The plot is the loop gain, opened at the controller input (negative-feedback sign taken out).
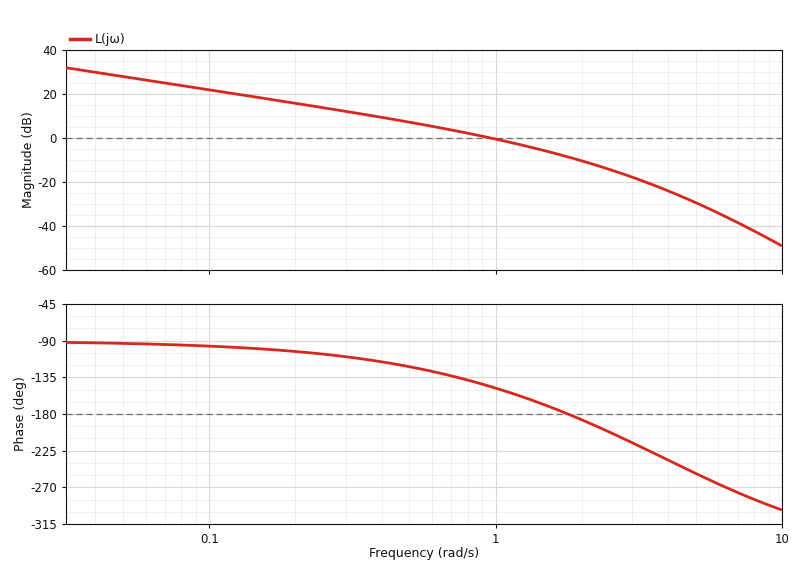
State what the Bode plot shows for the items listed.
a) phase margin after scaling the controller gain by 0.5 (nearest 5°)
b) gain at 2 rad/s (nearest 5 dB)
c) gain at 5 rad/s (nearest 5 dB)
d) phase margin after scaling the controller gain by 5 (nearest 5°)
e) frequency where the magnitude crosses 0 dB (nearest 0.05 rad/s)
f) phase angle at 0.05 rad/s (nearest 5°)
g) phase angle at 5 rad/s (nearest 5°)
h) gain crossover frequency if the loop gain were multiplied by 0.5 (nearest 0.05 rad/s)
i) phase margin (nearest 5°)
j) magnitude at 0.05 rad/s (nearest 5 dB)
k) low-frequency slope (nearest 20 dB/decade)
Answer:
55°
-10 dB
-30 dB
-20°
0.95 rad/s
-95°
-255°
0.55 rad/s
35°
30 dB
-20 dB/decade
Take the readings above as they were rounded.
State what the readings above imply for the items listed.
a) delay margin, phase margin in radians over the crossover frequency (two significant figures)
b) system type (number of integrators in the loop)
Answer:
0.64 s
1
